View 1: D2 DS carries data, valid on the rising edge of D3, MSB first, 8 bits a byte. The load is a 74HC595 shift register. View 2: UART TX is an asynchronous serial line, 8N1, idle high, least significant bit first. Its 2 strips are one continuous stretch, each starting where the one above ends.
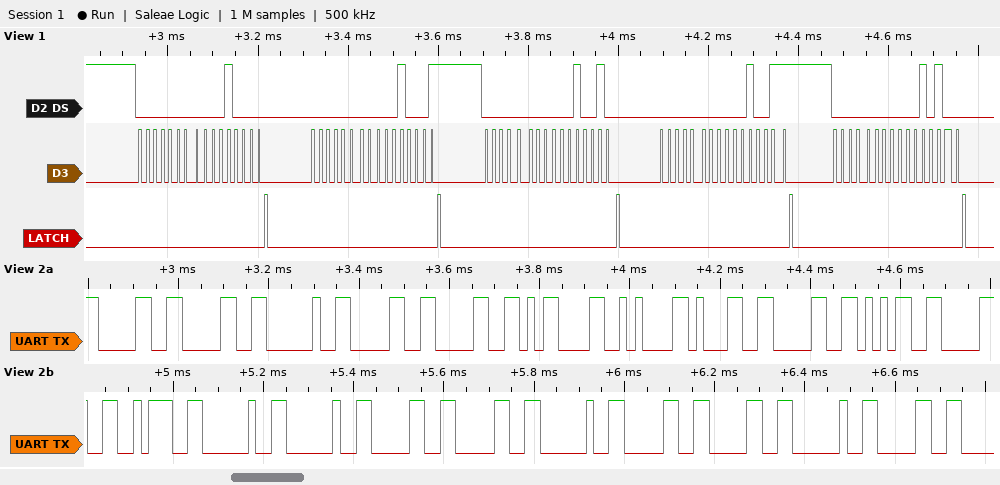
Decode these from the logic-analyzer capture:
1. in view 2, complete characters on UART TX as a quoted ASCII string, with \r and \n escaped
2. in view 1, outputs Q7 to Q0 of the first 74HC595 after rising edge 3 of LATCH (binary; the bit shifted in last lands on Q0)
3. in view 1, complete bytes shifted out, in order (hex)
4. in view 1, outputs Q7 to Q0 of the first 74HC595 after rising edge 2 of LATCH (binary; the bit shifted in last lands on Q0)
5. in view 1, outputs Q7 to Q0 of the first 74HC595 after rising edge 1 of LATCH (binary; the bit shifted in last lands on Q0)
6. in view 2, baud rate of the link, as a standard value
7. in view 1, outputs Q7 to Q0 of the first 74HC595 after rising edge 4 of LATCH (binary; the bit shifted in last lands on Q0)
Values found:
"00 00\r\n1050:  00 00 0"
00010010
00 10 00 11 00 12 00 13 00 14
00010001
00010000
57600 baud
00010011
